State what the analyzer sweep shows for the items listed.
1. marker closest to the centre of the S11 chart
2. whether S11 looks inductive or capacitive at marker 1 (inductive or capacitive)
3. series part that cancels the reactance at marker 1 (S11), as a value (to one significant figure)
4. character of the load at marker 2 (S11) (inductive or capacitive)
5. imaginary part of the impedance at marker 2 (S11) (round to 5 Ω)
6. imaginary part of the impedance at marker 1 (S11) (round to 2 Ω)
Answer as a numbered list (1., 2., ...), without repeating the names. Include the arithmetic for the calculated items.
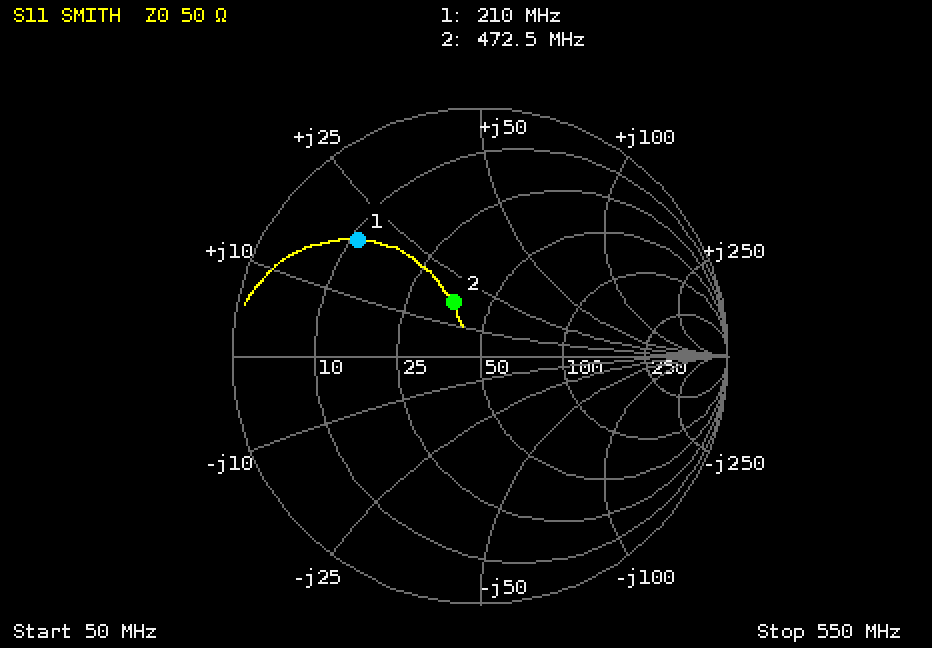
1. marker 2
2. inductive
3. C = 1/(2π × 210 MHz × 20 Ω) ≈ 37.9 pF, so 40 pF to one significant figure
4. inductive
5. +15 Ω
6. +20 Ω
